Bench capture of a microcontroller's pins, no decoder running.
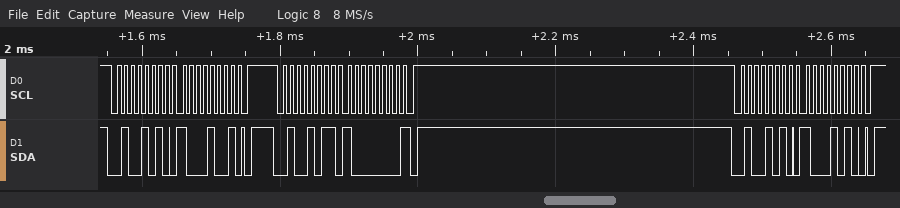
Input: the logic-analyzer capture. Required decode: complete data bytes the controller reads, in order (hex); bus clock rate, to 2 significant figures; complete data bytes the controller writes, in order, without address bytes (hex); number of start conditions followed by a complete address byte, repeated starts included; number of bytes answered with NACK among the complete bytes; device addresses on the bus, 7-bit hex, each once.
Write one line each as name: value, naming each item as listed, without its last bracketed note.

complete data bytes the controller reads, in order: 80
bus clock rate, to 2 significant figures: 100 kHz
complete data bytes the controller writes, in order, without address bytes: 89 8A
number of start conditions followed by a complete address byte, repeated starts included: 3
number of bytes answered with NACK among the complete bytes: 1
device addresses on the bus, 7-bit hex, each once: 0x25
